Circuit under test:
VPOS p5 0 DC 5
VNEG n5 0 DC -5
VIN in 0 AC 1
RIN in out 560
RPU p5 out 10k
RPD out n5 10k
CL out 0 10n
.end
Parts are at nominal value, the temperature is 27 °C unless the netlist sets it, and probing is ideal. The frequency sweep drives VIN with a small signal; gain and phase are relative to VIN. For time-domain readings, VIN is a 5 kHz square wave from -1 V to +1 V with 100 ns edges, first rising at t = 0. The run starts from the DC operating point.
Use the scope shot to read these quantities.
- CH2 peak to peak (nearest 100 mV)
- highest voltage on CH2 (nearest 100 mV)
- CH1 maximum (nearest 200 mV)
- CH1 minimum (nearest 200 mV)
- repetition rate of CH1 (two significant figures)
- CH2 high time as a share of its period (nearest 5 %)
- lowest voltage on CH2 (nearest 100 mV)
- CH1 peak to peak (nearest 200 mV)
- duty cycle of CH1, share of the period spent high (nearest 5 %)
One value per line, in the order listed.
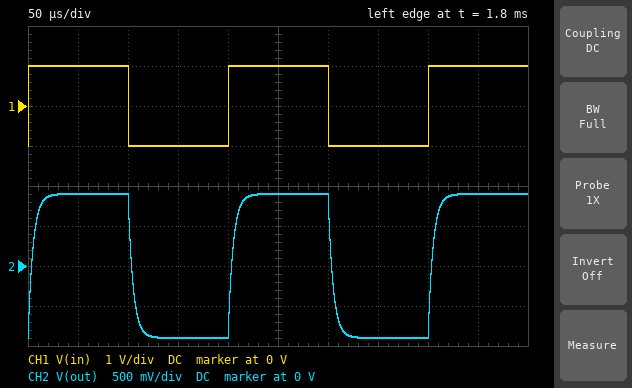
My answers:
1.8 V
900 mV
1.0 V
-1.0 V
5.0 kHz
50 %
-900 mV
2.0 V
50 %
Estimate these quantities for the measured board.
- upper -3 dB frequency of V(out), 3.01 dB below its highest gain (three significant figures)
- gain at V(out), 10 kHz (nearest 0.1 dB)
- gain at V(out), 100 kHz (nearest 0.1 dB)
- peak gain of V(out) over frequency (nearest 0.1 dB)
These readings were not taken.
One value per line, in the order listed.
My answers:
31.6 kHz
-1.3 dB
-11.3 dB
-0.9 dB
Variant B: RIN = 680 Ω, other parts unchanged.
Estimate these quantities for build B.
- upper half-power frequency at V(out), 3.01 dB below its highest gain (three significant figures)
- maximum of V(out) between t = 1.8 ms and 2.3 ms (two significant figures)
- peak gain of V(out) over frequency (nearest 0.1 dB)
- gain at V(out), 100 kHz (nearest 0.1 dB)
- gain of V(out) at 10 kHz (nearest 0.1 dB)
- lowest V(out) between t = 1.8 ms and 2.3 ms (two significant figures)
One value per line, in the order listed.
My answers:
26.6 kHz
880 mV
-1.1 dB
-12.9 dB
-1.7 dB
-880 mV
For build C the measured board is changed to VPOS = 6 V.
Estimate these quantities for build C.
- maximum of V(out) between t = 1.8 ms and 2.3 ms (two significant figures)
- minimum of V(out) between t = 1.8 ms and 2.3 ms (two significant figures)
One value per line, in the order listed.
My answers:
950 mV
-850 mV
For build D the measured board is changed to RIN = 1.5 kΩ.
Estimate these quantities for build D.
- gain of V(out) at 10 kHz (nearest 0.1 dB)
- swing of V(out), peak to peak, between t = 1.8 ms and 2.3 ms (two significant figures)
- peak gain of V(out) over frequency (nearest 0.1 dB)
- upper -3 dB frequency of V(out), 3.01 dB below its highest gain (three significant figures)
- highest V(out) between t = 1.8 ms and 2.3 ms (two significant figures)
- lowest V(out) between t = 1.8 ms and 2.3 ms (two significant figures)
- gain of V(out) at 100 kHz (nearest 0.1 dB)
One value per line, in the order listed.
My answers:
-4.1 dB
1.5 V
-2.3 dB
13.8 kHz
770 mV
-770 mV
-19.6 dB
